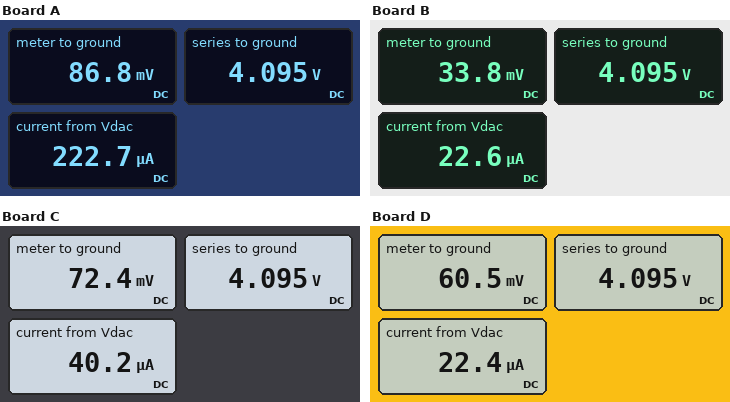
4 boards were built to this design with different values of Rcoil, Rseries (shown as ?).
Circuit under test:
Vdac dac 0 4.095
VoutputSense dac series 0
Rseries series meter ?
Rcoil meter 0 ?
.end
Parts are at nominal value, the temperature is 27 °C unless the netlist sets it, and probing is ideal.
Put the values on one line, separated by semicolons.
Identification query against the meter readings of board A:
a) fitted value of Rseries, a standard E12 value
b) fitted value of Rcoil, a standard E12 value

18 kΩ; 390 Ω
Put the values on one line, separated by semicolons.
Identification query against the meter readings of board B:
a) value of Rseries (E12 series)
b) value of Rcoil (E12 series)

180 kΩ; 1.5 kΩ
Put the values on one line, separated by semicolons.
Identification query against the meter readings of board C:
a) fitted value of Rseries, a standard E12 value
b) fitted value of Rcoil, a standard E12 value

100 kΩ; 1.8 kΩ
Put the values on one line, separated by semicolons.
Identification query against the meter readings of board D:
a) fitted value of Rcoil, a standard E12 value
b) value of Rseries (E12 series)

2.7 kΩ; 180 kΩ
